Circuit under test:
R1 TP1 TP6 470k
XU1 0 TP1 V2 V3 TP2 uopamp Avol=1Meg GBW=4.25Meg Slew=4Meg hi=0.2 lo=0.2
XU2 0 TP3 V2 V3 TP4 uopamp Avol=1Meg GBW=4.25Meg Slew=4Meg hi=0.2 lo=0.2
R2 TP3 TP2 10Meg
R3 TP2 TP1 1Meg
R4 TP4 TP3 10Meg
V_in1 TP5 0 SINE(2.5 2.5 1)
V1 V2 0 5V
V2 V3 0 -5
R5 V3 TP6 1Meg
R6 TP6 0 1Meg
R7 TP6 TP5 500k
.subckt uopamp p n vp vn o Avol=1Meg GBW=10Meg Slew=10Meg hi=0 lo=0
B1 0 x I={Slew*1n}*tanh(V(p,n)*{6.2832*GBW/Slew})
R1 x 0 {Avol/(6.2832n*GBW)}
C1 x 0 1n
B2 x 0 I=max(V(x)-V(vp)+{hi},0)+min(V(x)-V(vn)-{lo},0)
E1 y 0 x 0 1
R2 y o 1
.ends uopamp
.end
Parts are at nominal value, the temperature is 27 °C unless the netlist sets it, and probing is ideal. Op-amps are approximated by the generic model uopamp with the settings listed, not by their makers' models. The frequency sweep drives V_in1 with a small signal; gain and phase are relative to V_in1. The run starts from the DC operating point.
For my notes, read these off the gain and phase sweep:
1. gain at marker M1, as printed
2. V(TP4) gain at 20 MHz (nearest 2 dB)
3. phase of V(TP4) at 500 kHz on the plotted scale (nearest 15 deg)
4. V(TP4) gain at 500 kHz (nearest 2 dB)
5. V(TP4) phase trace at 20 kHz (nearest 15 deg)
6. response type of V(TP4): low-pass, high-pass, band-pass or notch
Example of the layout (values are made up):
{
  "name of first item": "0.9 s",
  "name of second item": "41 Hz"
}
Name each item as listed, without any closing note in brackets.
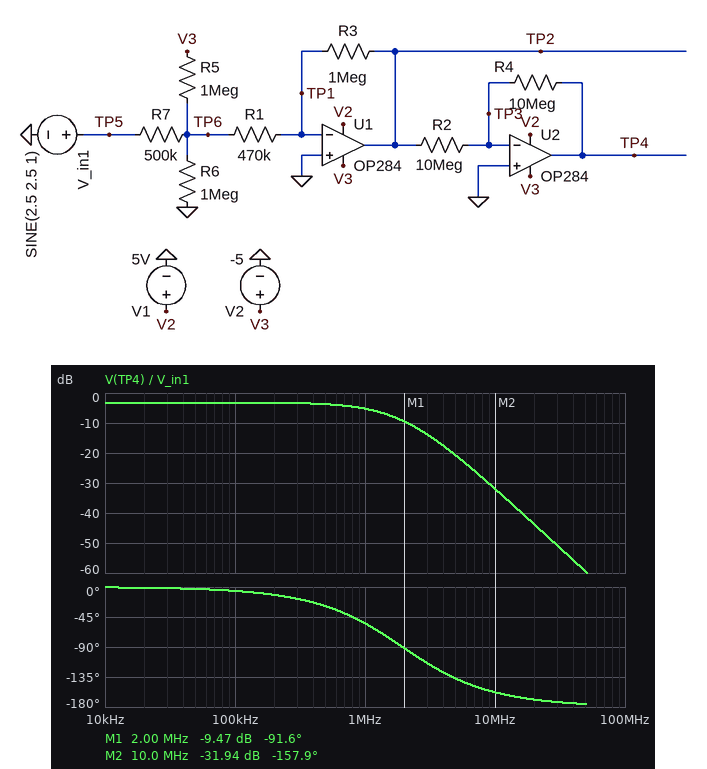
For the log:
{
  "gain at marker M1, as printed": "-9.47 dB",
  "V(TP4) gain at 20 MHz": "-44 dB",
  "phase of V(TP4) at 500 kHz on the plotted scale": "-30 deg",
  "V(TP4) gain at 500 kHz": "-4 dB",
  "V(TP4) phase trace at 20 kHz": "0 deg",
  "response type of V(TP4): low-pass, high-pass, band-pass or notch": "low-pass"
}
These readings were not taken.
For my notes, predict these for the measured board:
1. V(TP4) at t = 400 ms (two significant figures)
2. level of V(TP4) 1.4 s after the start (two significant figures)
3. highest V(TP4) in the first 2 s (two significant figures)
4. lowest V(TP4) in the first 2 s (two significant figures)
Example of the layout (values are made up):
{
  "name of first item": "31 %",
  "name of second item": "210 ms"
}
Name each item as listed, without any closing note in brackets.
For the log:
{
  "V(TP4) at t = 400 ms": "1.0 V",
  "level of V(TP4) 1.4 s after the start": "1.0 V",
  "highest V(TP4) in the first 2 s": "1.7 V",
  "lowest V(TP4) in the first 2 s": "-1.7 V"
}
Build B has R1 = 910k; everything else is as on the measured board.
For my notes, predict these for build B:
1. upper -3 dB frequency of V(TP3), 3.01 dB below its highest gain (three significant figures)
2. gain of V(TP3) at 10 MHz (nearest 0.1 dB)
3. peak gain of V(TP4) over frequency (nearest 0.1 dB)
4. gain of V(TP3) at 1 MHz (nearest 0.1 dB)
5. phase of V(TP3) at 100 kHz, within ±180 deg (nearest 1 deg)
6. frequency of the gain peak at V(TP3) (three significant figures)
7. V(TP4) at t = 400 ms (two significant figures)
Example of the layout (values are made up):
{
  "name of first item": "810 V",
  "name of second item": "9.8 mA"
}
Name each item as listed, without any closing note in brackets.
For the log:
{
  "upper -3 dB frequency of V(TP3), 3.01 dB below its highest gain": "5.32 MHz",
  "gain of V(TP3) at 10 MHz": "-26.6 dB",
  "peak gain of V(TP4) over frequency": "-7.3 dB",
  "gain of V(TP3) at 1 MHz": "-21.5 dB",
  "phase of V(TP3) at 100 kHz, within ±180 deg": "-95 deg",
  "frequency of the gain peak at V(TP3)": "2.20 MHz",
  "V(TP4) at t = 400 ms": "630 mV"
}
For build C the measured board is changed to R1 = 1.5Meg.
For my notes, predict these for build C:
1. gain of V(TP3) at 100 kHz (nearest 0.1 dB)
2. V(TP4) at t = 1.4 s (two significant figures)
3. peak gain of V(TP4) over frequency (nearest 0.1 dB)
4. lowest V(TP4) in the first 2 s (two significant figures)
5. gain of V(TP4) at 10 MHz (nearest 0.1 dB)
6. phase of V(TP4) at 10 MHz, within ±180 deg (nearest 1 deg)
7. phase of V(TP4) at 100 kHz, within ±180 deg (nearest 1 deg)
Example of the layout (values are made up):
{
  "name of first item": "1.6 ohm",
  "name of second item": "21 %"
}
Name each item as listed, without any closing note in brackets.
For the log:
{
  "gain of V(TP3) at 100 kHz": "-43.5 dB",
  "V(TP4) at t = 1.4 s": "420 mV",
  "peak gain of V(TP4) over frequency": "-10.9 dB",
  "lowest V(TP4) in the first 2 s": "-710 mV",
  "gain of V(TP4) at 10 MHz": "-36.2 dB",
  "phase of V(TP4) at 10 MHz, within ±180 deg": "-153 deg",
  "phase of V(TP4) at 100 kHz, within ±180 deg": "-5 deg"
}
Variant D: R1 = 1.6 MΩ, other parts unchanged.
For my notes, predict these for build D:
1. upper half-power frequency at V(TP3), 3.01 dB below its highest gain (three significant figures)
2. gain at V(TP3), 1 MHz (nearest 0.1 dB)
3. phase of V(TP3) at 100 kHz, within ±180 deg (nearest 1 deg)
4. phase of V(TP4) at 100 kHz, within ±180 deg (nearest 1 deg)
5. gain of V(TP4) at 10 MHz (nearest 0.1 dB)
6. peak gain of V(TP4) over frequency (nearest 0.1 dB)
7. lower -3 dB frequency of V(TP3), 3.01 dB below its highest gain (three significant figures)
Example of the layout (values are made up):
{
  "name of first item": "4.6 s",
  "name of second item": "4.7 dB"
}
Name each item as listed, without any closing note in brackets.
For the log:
{
  "upper half-power frequency at V(TP3), 3.01 dB below its highest gain": "5.88 MHz",
  "gain at V(TP3), 1 MHz": "-25.3 dB",
  "phase of V(TP3) at 100 kHz, within ±180 deg": "-95 deg",
  "phase of V(TP4) at 100 kHz, within ±180 deg": "-5 deg",
  "gain of V(TP4) at 10 MHz": "-36.5 dB",
  "peak gain of V(TP4) over frequency": "-11.4 dB",
  "lower -3 dB frequency of V(TP3), 3.01 dB below its highest gain": "997 kHz"
}
